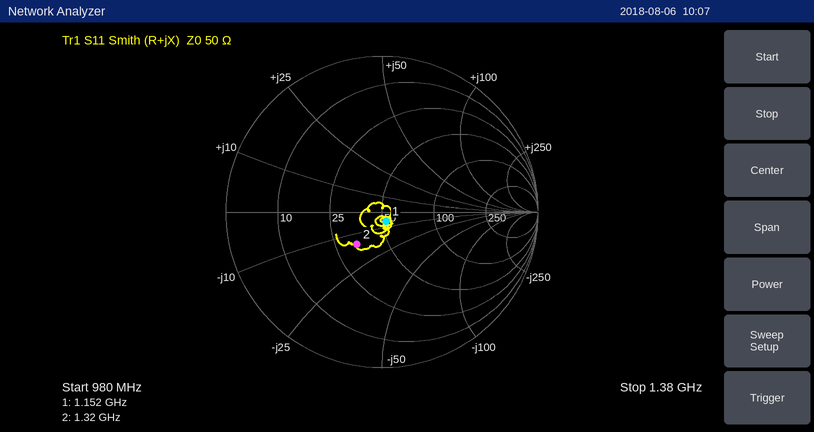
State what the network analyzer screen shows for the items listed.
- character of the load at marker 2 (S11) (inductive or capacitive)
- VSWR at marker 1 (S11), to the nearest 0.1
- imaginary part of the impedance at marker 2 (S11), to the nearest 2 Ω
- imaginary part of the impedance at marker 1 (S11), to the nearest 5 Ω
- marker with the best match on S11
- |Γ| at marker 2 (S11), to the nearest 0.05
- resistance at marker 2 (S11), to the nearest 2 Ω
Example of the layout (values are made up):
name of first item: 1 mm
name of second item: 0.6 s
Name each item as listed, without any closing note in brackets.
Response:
character of the load at marker 2 (S11): capacitive
VSWR at marker 1 (S11), to the nearest 0.1: 1.1
imaginary part of the impedance at marker 2 (S11), to the nearest 2 Ω: -14 Ω
imaginary part of the impedance at marker 1 (S11), to the nearest 5 Ω: -5 Ω
marker with the best match on S11: marker 1
|Γ| at marker 2 (S11), to the nearest 0.05: 0.25
resistance at marker 2 (S11), to the nearest 2 Ω: 34 Ω
